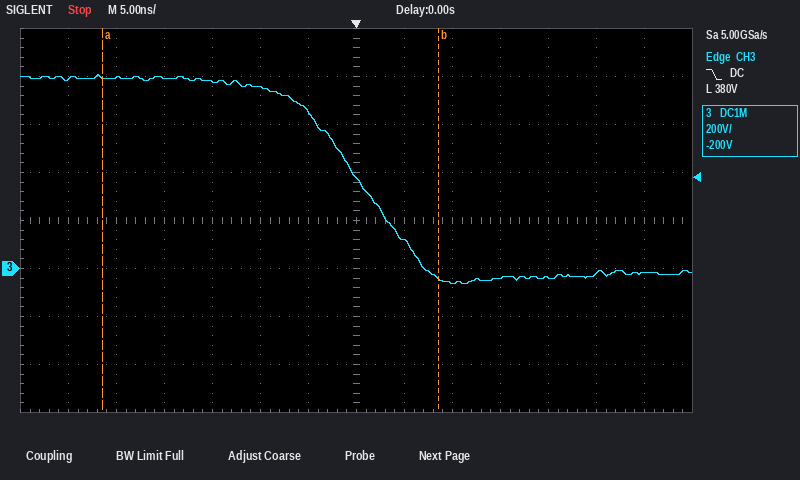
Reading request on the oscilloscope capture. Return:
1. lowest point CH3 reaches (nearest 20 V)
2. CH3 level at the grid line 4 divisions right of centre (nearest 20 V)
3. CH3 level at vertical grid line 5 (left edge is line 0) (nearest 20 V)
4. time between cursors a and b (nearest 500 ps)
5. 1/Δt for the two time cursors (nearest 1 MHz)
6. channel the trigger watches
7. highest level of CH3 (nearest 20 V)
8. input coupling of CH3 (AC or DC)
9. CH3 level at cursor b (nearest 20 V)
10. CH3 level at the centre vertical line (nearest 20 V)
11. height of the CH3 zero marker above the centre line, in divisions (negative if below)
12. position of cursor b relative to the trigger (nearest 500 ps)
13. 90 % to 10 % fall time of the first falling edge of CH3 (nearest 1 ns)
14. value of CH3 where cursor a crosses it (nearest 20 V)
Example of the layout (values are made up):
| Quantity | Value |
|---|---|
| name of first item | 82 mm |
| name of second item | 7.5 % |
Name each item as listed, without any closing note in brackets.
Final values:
| Quantity | Value |
|---|---|
| lowest point CH3 reaches | -60 V |
| CH3 level at the grid line 4 divisions right of centre | -40 V |
| CH3 level at vertical grid line 5 (left edge is line 0) | 760 V |
| time between cursors a and b | 35.0 ns |
| 1/Δt for the two time cursors | 29 MHz |
| channel the trigger watches | CH3 |
| highest level of CH3 | 800 V |
| input coupling of CH3 | DC |
| CH3 level at cursor b | -40 V |
| CH3 level at the centre vertical line | 380 V |
| height of the CH3 zero marker above the centre line, in divisions | -1.0 div |
| position of cursor b relative to the trigger | +8.5 ns |
| 90 % to 10 % fall time of the first falling edge of CH3 | 13 ns |
| value of CH3 where cursor a crosses it | 800 V |
